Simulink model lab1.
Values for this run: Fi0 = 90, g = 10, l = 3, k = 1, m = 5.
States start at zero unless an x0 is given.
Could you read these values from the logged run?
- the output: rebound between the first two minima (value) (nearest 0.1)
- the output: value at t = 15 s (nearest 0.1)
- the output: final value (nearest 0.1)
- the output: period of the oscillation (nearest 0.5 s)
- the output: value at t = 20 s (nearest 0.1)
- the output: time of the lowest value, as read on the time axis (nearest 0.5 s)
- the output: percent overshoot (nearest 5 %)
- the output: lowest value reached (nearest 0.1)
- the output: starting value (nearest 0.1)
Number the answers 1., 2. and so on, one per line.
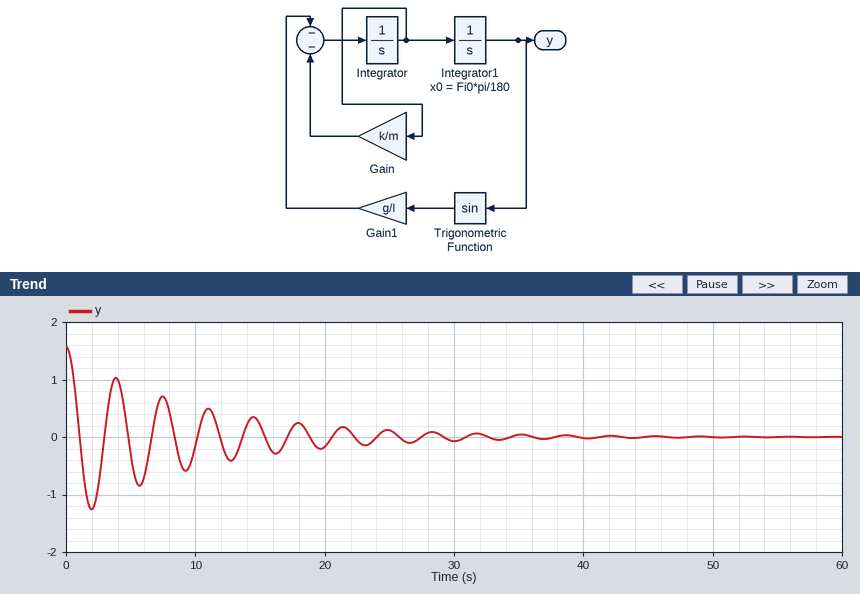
1. 1.0
2. 0.2
3. 0.0
4. 3.5 s
5. -0.2
6. 2.0 s
7. 80 %
8. -1.3
9. 1.6
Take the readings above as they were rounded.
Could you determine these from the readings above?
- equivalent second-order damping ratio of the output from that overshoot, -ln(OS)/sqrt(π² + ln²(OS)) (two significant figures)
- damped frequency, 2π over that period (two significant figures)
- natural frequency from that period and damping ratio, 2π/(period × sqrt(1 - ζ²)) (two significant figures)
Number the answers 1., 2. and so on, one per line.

1. 0.071
2. 1.8 rad/s
3. 1.8 rad/s
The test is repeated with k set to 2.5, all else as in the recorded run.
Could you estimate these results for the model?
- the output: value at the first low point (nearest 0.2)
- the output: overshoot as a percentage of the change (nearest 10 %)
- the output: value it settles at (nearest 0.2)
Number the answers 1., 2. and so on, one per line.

1. -1.0
2. 60 %
3. 0.0
